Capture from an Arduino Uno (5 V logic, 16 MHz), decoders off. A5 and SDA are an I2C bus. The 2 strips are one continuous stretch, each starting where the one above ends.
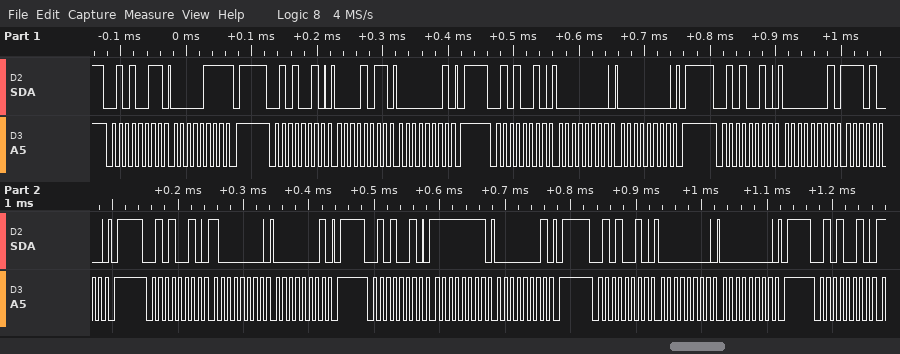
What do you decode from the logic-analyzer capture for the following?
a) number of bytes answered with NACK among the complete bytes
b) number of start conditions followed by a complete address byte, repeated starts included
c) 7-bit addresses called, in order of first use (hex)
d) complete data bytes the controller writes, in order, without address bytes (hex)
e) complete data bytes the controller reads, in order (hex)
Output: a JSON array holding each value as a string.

["1", "8", "0x29", "0B 01 00 00 01 E8 80 01 FF 01 00 00", "07"]
